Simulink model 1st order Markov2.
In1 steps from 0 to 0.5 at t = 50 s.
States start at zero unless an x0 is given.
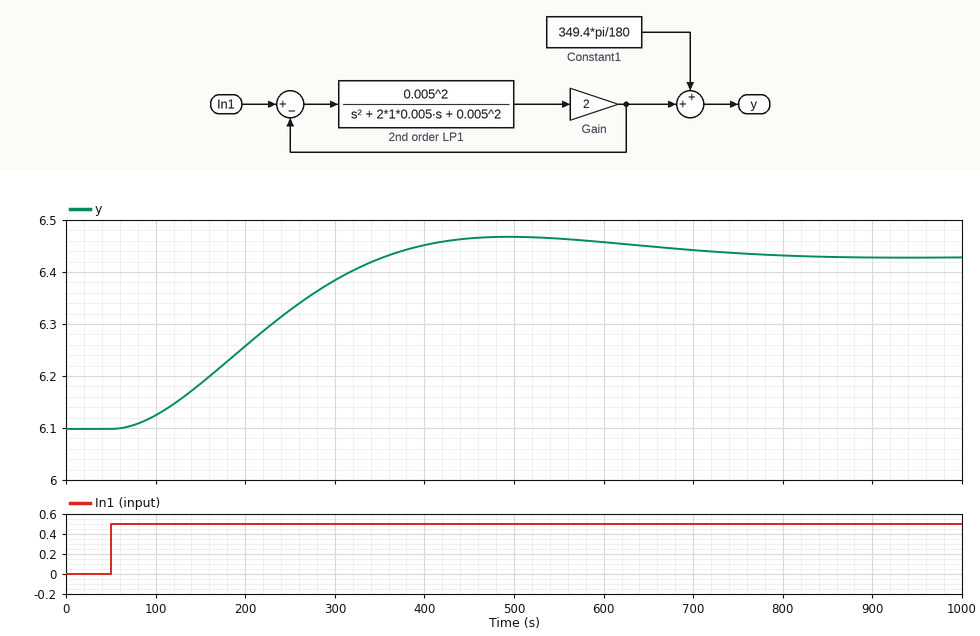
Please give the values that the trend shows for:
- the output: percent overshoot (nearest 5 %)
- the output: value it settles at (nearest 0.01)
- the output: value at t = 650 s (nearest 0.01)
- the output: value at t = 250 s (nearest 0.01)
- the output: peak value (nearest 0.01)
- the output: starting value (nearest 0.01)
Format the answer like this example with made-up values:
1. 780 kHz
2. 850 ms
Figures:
1. 10 %
2. 6.43
3. 6.45
4. 6.33
5. 6.47
6. 6.10
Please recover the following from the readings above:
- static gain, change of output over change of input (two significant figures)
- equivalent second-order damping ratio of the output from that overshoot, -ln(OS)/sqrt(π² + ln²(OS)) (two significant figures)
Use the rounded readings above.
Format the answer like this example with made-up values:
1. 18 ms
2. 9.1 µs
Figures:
1. 0.66
2. 0.59
